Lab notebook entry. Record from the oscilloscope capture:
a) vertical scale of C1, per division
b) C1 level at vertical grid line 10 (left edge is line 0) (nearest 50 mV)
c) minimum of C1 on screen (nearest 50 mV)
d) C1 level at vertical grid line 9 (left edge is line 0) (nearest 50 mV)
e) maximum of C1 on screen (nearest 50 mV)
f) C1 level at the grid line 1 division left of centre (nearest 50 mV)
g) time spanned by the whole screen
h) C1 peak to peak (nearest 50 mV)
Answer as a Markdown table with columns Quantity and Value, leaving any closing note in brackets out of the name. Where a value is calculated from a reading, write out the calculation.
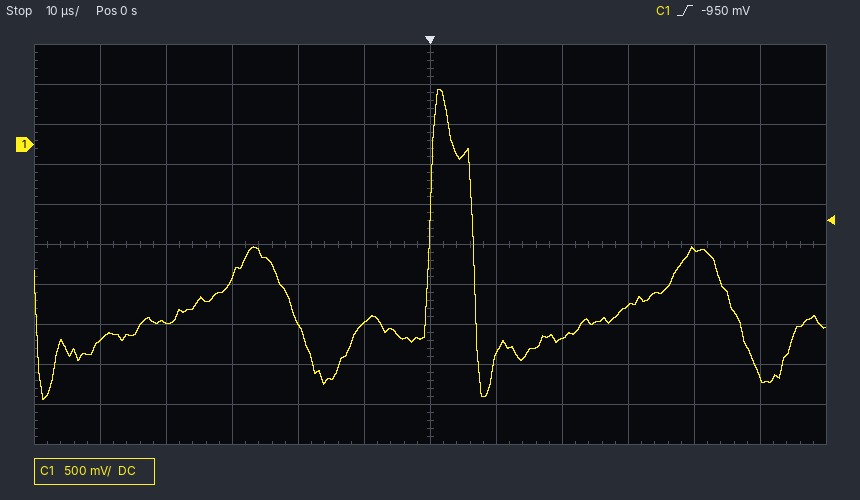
| Quantity | Value |
|---|---|
| vertical scale of C1, per division | 500 mV |
| C1 level at vertical grid line 10 (left edge is line 0) | -1.30 V |
| minimum of C1 on screen | -3.20 V |
| C1 level at vertical grid line 9 (left edge is line 0) | -2.00 V |
| maximum of C1 on screen | 700 mV |
| C1 level at the grid line 1 division left of centre | -2.25 V |
| time spanned by the whole screen | 120 µs |
| C1 peak to peak | 700 mV − (-3.20 V) = 3.90 V |
